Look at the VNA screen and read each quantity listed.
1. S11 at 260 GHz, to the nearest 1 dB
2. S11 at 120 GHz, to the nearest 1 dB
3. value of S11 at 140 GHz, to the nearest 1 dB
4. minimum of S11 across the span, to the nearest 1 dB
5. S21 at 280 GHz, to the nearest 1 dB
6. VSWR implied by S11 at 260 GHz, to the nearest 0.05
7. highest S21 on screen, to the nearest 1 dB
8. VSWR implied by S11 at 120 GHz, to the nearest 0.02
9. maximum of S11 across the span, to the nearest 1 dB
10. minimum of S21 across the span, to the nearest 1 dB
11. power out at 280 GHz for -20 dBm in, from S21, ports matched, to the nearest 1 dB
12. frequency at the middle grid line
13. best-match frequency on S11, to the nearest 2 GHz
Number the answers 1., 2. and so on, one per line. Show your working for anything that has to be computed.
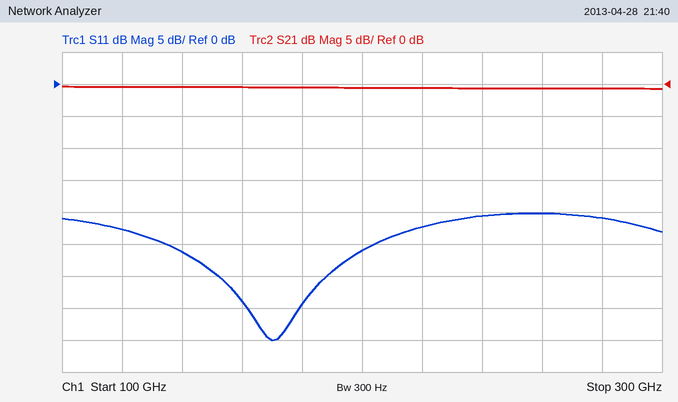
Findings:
1. -20 dB
2. -23 dB
3. -26 dB
4. -40 dB
5. -1 dB
6. |Γ| = 10^(-20/20) = 0.1000; VSWR = (1 + 0.1000)/(1 − 0.1000) ≈ 1.22, so 1.20 to the nearest 0.05
7. 0 dB
8. |Γ| = 10^(-23/20) = 0.0708; VSWR = (1 + 0.0708)/(1 − 0.0708) ≈ 1.15, so 1.16 to the nearest 0.02
9. -20 dB
10. -1 dB
11. -20 dBm + (-1 dB) = -21 dBm
12. 200 GHz
13. 170 GHz
